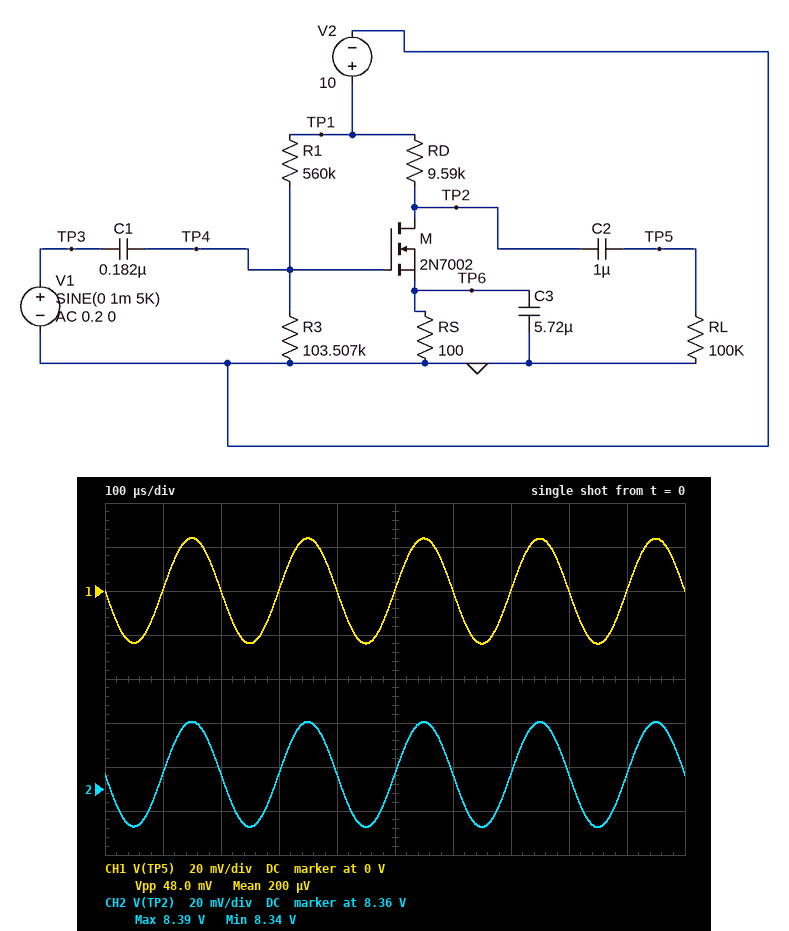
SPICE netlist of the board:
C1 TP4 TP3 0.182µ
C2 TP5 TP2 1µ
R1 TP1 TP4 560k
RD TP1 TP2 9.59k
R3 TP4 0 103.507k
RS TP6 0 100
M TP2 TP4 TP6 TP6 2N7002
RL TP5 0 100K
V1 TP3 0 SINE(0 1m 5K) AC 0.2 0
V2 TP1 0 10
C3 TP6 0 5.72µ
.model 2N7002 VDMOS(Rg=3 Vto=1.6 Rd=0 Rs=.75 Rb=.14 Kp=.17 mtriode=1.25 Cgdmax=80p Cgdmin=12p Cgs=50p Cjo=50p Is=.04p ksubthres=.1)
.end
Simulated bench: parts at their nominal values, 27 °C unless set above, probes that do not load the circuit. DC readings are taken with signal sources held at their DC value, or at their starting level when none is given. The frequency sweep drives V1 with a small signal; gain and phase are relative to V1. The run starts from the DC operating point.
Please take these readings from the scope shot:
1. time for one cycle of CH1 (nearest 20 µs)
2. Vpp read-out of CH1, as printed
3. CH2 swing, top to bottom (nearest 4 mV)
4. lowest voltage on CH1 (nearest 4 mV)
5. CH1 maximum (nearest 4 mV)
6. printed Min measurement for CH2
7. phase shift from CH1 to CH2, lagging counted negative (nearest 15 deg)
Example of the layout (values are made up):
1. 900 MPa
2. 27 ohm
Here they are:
1. 200 µs
2. 48.0 mV
3. 48 mV
4. -24 mV
5. 24 mV
6. 8.34 V
7. 0 deg
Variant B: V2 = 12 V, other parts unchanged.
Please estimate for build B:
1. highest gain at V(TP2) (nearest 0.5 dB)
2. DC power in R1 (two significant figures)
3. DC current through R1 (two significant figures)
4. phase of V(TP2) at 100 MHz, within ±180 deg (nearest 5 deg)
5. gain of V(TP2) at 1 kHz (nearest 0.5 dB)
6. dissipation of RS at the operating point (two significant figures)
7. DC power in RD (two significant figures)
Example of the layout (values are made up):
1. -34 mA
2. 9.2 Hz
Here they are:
1. -5.0 dB
2. 180 µW
3. 18 µA
4. 15 deg
5. -11.0 dB
6. 150 µW
7. 15 mW
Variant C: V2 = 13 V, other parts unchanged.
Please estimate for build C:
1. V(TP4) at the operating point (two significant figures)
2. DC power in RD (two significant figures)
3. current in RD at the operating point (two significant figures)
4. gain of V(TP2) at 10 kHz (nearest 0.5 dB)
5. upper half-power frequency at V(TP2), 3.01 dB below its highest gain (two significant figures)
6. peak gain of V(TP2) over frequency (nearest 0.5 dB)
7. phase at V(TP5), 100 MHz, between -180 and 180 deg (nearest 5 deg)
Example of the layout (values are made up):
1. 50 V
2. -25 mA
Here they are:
1. 2.0 V
2. 17 mW
3. 1.3 mA
4. -22.0 dB
5. 800 MHz
6. -5.5 dB
7. 30 deg
